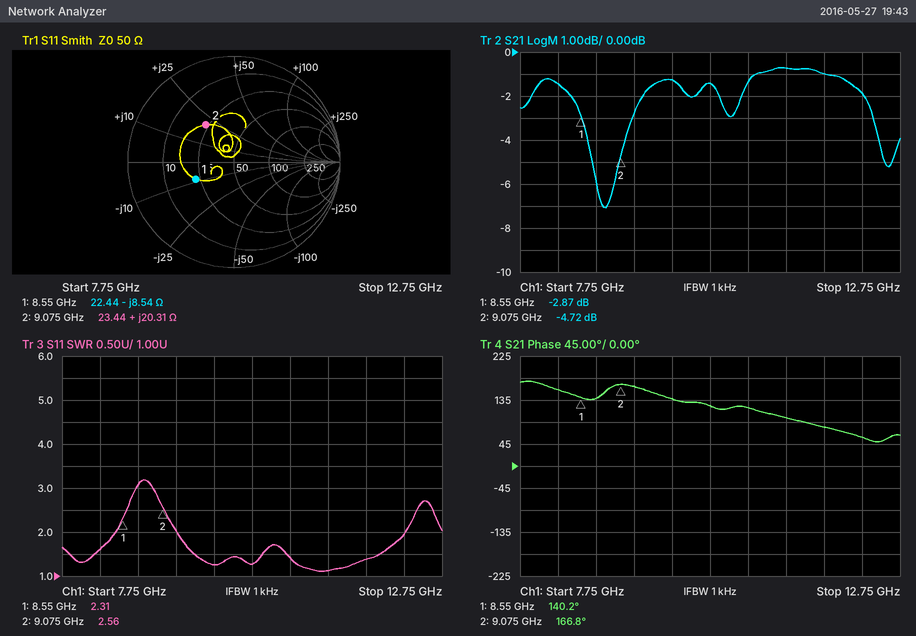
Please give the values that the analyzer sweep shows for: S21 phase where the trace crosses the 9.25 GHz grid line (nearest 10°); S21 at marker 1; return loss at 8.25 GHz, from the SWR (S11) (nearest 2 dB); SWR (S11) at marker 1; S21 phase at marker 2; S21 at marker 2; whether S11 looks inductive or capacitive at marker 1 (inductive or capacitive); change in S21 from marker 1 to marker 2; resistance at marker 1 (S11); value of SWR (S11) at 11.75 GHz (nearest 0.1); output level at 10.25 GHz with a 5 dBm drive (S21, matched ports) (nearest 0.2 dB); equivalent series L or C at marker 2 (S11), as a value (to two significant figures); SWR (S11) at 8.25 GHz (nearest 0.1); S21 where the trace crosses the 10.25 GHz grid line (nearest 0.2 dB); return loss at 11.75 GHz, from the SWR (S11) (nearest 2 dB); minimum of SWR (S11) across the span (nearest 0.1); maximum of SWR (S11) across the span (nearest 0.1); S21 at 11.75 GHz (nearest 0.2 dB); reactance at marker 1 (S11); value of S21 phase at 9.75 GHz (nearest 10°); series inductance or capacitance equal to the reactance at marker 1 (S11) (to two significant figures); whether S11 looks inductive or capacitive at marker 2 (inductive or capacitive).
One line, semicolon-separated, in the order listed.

160°; -2.87 dB; 12 dB; 2.31; 166.8°; -4.72 dB; capacitive; -1.85 dB; 22.44 Ω; 1.4; 3.6 dBm; 360 pH; 1.6; -1.4 dB; 16 dB; 1.1; 3.2; -1.0 dB; -8.54 Ω; 140°; 2.2 pF; inductive
